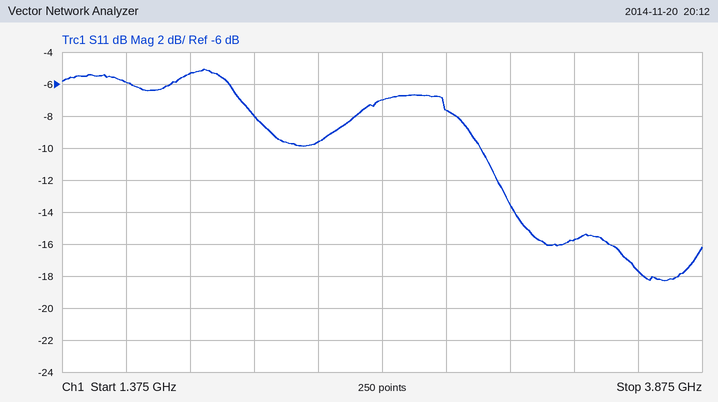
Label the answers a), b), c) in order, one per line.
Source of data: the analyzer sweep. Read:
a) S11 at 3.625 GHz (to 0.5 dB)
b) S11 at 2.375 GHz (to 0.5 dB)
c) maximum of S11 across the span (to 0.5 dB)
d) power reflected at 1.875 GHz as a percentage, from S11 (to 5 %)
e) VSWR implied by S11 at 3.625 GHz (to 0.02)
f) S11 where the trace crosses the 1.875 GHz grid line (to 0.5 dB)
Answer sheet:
a) -17.5 dB
b) -9.5 dB
c) -5.0 dB
d) 30 %
e) 1.30
f) -5.5 dB
